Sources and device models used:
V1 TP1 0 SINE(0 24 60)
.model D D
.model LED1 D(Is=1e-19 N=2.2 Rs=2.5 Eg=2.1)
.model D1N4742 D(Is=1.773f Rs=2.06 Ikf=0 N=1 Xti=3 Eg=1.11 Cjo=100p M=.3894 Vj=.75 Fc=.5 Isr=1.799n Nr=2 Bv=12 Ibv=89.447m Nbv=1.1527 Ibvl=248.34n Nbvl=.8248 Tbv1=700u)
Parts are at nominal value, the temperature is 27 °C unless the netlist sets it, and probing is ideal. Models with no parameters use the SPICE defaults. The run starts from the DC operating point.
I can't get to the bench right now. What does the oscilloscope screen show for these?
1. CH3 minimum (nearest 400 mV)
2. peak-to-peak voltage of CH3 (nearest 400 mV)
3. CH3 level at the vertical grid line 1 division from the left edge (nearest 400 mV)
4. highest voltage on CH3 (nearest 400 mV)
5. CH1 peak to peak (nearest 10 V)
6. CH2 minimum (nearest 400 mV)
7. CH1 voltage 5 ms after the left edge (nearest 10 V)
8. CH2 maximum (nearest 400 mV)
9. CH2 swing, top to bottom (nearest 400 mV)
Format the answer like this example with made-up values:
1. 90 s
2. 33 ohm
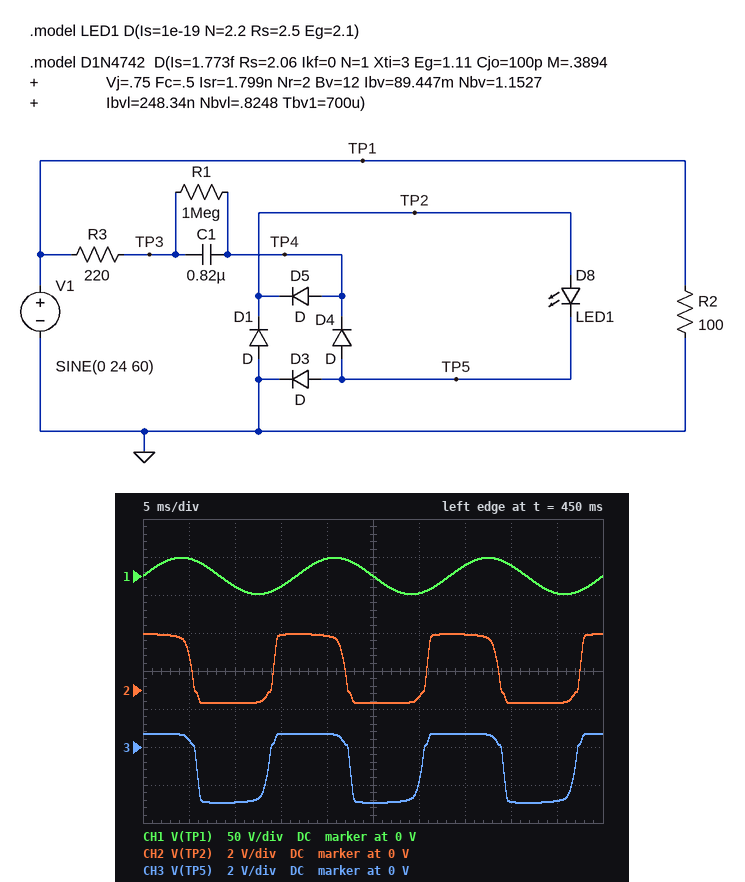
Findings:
1. -2.8 V
2. 3.6 V
3. 400 mV
4. 800 mV
5. 50 V
6. -800 mV
7. 20 V
8. 2.8 V
9. 3.6 V
